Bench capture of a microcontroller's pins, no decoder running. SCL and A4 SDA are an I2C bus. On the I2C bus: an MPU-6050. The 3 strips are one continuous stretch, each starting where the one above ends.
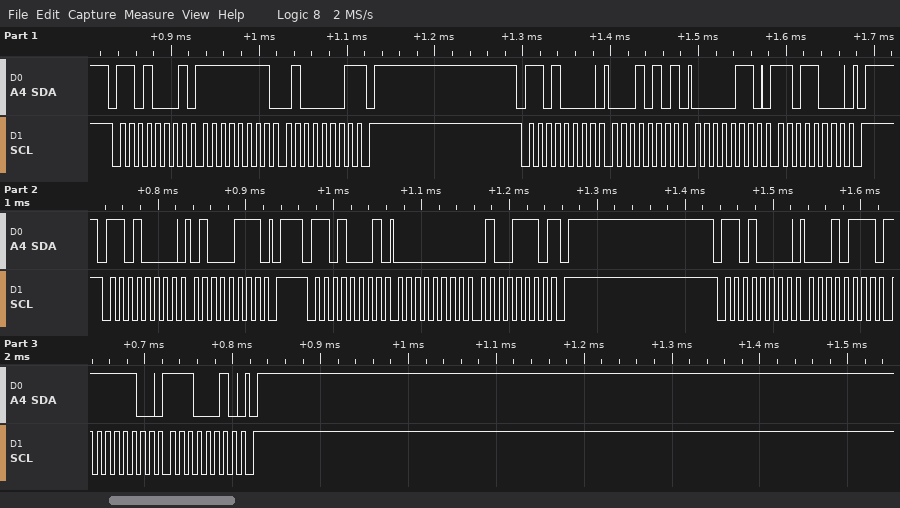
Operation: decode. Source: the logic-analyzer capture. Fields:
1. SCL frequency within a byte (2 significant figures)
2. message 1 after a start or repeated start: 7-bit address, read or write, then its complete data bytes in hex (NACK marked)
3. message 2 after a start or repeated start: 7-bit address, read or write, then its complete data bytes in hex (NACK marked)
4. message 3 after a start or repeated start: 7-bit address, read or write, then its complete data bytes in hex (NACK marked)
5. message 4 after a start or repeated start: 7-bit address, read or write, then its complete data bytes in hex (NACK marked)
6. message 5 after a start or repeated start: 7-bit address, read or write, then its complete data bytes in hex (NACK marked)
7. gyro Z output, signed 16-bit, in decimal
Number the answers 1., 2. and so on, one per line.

1. 100 kHz
2. 0x68 read: FF 41 NACK
3. 0x68 write: 15 06 D8
4. 0x68 write: 47
5. 0x68 read: 00 4E NACK
6. 0x68 write: 17 FC E2
7. 78
